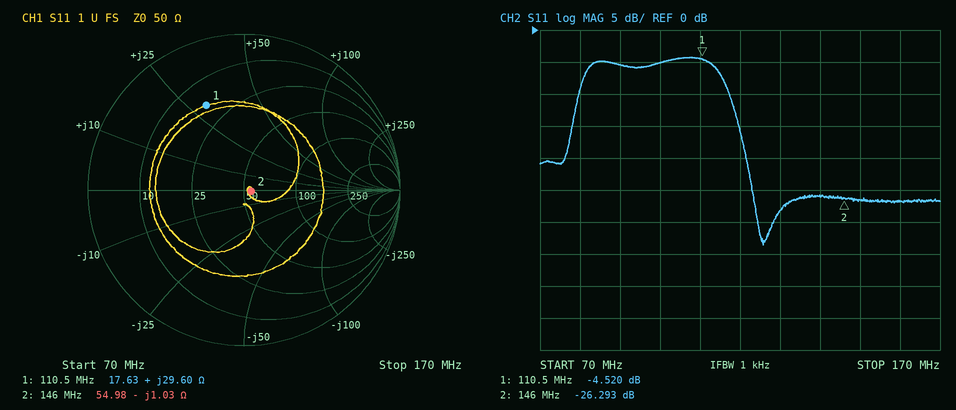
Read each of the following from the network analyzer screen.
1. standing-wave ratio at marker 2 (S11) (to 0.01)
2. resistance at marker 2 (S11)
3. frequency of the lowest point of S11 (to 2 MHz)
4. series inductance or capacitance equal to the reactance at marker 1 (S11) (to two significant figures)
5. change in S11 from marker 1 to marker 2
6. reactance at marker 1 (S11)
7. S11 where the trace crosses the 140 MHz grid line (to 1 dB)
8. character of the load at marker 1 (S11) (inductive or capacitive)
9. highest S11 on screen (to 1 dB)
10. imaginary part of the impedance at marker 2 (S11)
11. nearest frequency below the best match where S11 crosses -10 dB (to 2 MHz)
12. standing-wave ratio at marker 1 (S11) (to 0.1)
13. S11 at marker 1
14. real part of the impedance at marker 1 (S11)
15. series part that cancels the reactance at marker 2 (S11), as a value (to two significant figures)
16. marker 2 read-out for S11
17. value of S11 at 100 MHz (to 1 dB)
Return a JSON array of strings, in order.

["1.10", "54.98 Ω", "126 MHz", "43 nH", "-21.773 dB", "+29.60 Ω", "-26 dB", "inductive", "-4 dB", "-1.03 Ω", "118 MHz", "3.9", "-4.520 dB", "17.63 Ω", "1.1 nH", "-26.293 dB", "-5 dB"]
